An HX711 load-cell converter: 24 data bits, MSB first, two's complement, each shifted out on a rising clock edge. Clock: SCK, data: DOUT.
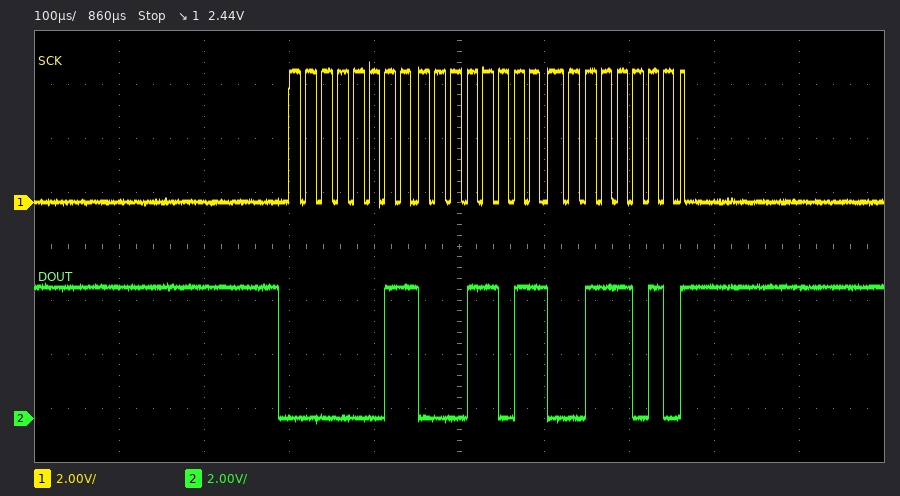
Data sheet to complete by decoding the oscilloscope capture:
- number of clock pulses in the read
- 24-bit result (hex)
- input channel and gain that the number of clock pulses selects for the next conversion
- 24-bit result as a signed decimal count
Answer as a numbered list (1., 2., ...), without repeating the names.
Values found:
1. 25
2. 0x031B3A
3. channel A, gain 128
4. 203578
